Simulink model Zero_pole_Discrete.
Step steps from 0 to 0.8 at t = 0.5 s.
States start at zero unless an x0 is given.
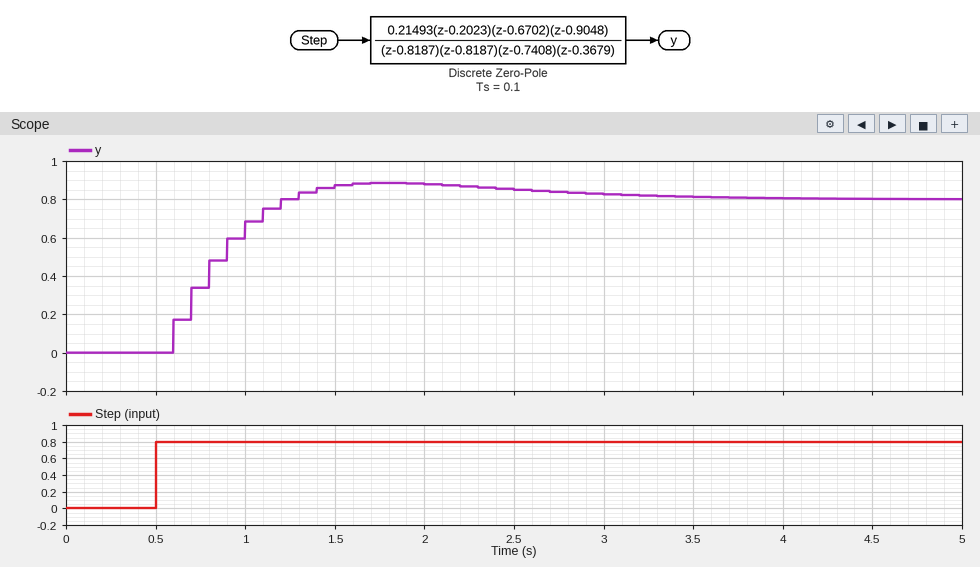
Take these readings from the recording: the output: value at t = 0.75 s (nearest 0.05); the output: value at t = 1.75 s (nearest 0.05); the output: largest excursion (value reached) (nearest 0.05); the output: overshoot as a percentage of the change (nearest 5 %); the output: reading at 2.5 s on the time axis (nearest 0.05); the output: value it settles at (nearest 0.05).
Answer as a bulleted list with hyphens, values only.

- 0.35
- 0.90
- 0.90
- 10 %
- 0.85
- 0.80
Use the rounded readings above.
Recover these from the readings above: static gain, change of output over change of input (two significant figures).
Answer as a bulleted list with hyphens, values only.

- 1.0
